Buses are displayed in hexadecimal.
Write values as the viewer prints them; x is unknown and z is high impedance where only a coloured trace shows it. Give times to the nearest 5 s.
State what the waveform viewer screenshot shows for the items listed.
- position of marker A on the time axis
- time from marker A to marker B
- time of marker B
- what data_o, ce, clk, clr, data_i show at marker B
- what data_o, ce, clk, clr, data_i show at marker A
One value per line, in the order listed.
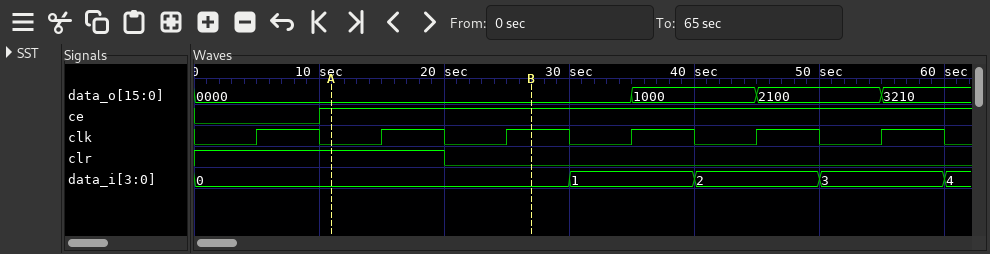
10 s
15 s
25 s
data_o=0000, ce=1, clk=1, clr=0, data_i=0
data_o=0000, ce=1, clk=0, clr=1, data_i=0
